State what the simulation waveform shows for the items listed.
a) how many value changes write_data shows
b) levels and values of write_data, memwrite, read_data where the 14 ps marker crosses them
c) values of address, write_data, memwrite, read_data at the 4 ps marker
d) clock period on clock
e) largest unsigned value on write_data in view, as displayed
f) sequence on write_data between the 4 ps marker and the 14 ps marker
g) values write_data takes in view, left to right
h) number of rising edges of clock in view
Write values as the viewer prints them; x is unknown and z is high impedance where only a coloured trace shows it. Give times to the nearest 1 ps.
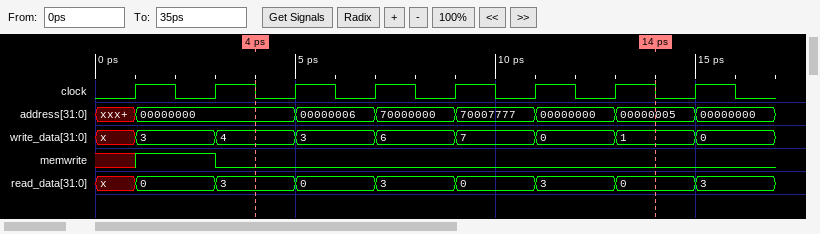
8
write_data=1, memwrite=0, read_data=0
address=00000000, write_data=4, memwrite=0, read_data=3
2 ps
7
4, 3, 6, 7, 0, 1
x, 3, 4, 3, 6, 7, 0, 1, 0
8
